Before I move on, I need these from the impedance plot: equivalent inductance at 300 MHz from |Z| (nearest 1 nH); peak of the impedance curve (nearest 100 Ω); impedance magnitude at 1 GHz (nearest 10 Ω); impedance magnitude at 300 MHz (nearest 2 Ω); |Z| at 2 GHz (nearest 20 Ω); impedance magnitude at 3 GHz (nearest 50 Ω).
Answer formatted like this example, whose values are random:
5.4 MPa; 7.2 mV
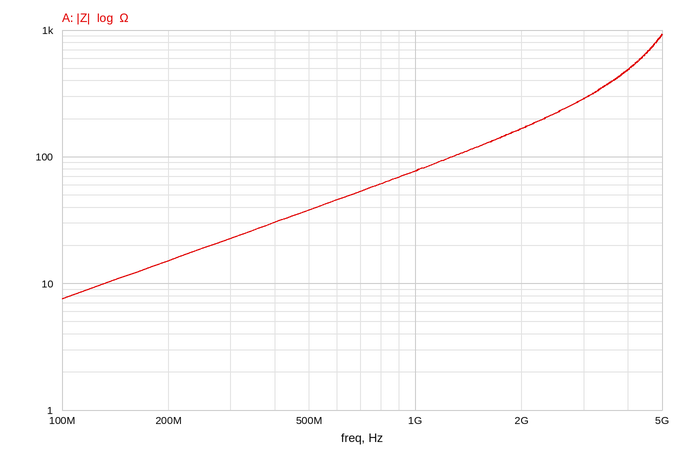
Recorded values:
12 nH; 900 Ω; 80 Ω; 22 Ω; 160 Ω; 300 Ω
